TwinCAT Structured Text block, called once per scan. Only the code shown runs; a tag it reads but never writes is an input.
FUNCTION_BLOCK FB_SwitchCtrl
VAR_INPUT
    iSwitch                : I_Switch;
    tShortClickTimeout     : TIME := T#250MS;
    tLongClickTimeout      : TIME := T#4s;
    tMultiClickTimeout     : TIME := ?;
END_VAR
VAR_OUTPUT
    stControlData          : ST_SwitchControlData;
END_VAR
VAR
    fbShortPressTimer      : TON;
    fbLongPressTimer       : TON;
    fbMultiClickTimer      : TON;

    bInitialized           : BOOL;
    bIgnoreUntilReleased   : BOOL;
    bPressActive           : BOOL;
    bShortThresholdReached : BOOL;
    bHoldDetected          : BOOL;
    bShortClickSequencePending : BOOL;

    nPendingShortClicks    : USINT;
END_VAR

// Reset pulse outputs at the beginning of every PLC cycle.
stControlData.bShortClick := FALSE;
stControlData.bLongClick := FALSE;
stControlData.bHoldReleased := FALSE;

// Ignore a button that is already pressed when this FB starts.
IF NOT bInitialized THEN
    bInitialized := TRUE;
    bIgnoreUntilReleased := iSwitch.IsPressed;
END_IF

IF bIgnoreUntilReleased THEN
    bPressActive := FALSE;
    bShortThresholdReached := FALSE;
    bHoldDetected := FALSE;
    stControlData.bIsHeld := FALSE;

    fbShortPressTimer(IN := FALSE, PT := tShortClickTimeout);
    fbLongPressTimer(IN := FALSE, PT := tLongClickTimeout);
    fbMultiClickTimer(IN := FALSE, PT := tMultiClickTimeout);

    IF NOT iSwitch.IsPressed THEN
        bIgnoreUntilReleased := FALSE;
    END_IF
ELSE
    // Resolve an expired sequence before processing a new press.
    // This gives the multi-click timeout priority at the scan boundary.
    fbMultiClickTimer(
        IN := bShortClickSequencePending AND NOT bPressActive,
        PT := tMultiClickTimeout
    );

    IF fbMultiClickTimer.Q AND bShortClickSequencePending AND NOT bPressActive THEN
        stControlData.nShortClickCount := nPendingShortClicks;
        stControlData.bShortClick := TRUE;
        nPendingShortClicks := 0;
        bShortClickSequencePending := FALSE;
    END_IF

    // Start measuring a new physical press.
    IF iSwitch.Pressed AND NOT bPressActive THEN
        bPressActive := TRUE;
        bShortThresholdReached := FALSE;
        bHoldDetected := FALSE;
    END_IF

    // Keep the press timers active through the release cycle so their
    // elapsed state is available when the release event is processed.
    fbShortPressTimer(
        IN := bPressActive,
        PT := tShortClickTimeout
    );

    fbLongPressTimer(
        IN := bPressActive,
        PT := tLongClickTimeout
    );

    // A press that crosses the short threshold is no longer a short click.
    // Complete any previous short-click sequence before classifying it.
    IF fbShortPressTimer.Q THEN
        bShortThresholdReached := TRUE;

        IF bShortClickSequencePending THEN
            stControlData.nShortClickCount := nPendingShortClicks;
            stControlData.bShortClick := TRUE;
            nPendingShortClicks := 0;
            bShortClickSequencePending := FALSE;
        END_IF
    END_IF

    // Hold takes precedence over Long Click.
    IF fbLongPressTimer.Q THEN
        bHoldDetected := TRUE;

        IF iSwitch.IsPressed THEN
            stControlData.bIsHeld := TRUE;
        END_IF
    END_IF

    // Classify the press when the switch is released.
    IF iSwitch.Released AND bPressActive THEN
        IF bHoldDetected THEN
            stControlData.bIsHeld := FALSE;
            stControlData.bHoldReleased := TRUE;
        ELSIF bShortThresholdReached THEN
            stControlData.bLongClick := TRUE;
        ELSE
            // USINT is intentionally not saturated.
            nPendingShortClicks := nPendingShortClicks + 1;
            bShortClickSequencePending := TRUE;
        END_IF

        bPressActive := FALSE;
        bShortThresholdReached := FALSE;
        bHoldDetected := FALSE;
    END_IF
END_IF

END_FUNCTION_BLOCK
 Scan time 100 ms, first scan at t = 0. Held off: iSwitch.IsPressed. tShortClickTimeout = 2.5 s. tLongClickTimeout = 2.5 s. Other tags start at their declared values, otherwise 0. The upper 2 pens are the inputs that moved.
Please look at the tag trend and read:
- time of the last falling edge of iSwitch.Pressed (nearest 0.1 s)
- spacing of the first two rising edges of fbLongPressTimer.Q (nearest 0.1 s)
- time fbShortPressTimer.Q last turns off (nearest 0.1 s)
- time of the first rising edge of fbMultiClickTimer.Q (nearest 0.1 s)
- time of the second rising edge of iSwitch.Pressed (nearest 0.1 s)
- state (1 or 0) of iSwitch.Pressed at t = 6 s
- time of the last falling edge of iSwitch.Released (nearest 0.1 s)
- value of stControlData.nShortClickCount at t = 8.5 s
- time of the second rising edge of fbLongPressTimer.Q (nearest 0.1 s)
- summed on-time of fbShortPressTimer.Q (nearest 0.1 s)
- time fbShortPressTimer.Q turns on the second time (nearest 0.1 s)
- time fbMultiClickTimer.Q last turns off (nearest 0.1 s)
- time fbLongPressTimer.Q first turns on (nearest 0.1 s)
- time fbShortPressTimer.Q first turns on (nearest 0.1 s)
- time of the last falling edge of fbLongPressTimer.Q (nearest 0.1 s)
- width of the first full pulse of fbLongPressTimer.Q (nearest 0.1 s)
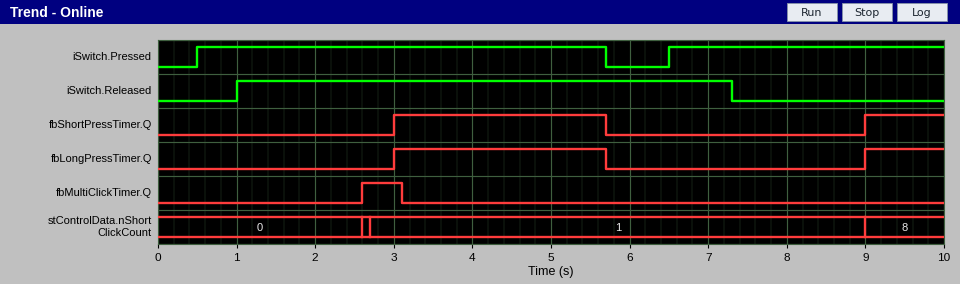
5.7 s
6.0 s
5.7 s
2.6 s
6.5 s
0
7.3 s
1
9.0 s
3.7 s
9.0 s
3.1 s
3.0 s
3.0 s
5.7 s
2.7 s
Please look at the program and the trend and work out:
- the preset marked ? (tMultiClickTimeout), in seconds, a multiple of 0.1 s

1.5 s
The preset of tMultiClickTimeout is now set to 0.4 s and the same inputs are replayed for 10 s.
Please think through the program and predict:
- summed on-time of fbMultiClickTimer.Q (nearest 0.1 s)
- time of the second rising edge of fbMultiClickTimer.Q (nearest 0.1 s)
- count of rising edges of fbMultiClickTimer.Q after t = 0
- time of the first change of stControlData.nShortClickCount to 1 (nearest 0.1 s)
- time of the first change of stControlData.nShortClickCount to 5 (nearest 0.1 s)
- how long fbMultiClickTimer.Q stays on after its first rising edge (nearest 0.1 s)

2.0 s
7.0 s
2
1.6 s
1.5 s
1.6 s
